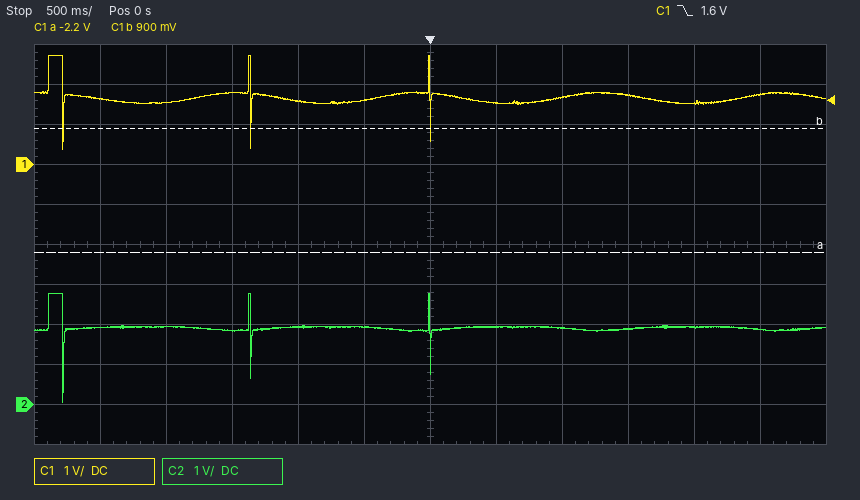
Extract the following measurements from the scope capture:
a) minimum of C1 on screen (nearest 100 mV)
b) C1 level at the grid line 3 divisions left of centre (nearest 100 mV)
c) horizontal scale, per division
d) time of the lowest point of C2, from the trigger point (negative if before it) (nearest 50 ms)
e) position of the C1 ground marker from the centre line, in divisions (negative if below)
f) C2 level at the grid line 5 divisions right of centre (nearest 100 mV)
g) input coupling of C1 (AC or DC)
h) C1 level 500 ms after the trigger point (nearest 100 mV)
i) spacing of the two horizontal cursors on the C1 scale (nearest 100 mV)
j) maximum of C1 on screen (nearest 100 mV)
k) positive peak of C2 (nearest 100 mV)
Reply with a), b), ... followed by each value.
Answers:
a) 400 mV
b) 1.8 V
c) 500 ms
d) -2.80 s
e) +2.0 div
f) 1.9 V
g) DC
h) 1.5 V
i) 3.1 V
j) 2.7 V
k) 2.8 V
